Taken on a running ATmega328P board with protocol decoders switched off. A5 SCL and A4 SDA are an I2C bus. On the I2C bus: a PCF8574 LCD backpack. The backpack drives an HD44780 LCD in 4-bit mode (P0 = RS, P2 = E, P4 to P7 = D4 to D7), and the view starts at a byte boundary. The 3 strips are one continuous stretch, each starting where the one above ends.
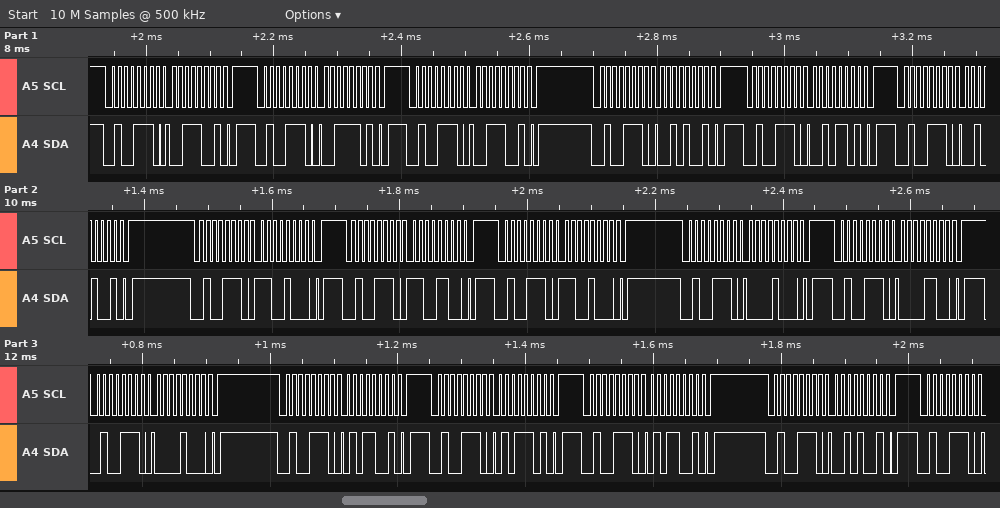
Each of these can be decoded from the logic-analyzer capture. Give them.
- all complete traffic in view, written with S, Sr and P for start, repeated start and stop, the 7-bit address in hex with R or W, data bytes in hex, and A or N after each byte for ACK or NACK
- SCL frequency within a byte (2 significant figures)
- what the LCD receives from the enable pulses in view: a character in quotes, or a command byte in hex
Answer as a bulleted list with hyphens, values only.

- S 27W A 39 A P S 27W A 3D A P S 27W A 39 A P S 27W A 29 A P S 27W A 2D A P S 27W A 29 A P S 27W A C8 A P S 27W A CC A P S 27W A C8 A P S 27W A 08 A P S 27W A 0C A P S 27W A 08 A P S 27W A 59 A P S 27W A 5D A P S 27W A 59 A P S 27W A 29 A P S 27W A
- 100 kHz
- '2' 0xC0
